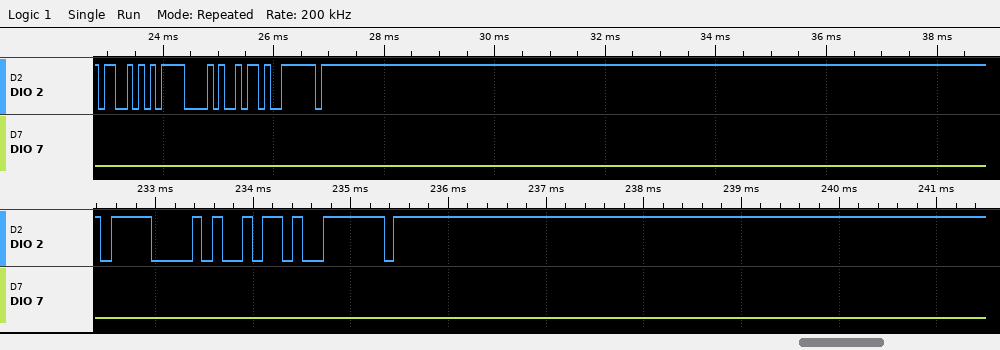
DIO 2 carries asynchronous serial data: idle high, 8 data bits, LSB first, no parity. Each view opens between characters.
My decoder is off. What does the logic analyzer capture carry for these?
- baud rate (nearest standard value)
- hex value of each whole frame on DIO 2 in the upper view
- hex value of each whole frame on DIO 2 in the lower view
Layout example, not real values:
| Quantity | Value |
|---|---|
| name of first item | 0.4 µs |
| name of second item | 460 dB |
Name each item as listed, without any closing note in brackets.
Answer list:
| Quantity | Value |
|---|---|
| baud rate | 9600 baud |
| hex value of each whole frame on DIO 2 in the upper view | 53, 0F, 69, 7E |
| hex value of each whole frame on DIO 2 in the lower view | 0F, 69, 7E |
